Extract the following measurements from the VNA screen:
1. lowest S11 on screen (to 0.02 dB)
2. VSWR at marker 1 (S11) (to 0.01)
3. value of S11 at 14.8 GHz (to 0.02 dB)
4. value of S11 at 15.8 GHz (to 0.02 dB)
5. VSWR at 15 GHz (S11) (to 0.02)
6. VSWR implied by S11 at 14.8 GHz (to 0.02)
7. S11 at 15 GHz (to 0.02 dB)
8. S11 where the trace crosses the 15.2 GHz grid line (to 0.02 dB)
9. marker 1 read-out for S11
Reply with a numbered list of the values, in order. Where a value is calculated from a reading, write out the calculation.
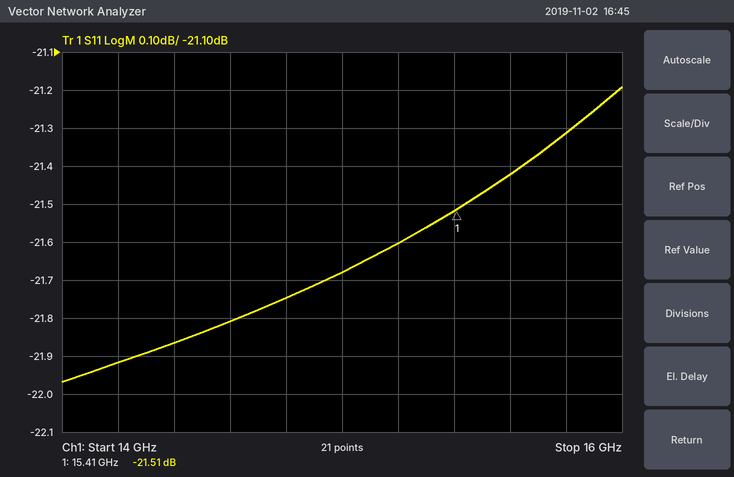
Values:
1. -21.96 dB
2. (1 + 0.0840)/(1 − 0.0840) ≈ 1.18
3. -21.74 dB
4. -21.32 dB
5. |Γ| = 10^(-21.68/20) = 0.0824; VSWR = (1 + 0.0824)/(1 − 0.0824) ≈ 1.18
6. |Γ| = 10^(-21.74/20) = 0.0818; VSWR = (1 + 0.0818)/(1 − 0.0818) ≈ 1.18
7. -21.68 dB
8. -21.60 dB
9. -21.51 dB
